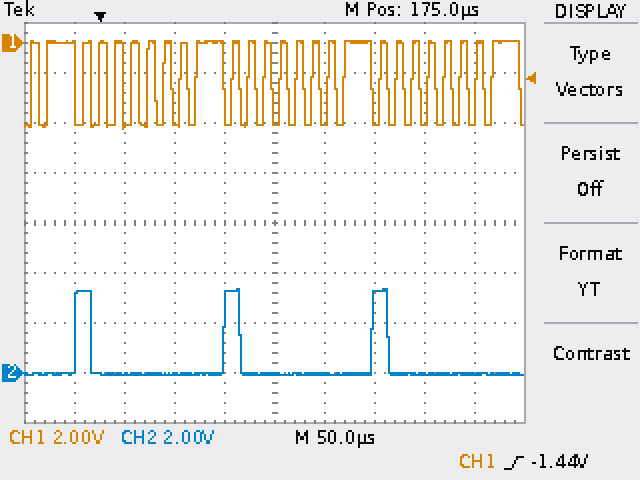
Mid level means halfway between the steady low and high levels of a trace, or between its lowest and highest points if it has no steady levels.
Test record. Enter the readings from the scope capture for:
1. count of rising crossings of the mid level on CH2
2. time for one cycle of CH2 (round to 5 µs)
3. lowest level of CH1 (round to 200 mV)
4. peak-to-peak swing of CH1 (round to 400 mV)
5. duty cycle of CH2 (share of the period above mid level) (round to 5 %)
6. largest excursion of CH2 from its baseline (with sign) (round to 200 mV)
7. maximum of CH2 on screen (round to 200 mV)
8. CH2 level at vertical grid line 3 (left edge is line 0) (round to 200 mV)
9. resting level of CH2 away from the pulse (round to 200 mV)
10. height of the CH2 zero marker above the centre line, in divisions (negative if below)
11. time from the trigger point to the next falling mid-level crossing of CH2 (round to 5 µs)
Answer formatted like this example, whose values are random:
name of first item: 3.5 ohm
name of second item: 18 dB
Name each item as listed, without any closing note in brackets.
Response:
count of rising crossings of the mid level on CH2: 3
time for one cycle of CH2: 150 µs
lowest level of CH1: -3.4 V
peak-to-peak swing of CH1: 3.6 V
duty cycle of CH2 (share of the period above mid level): 10 %
largest excursion of CH2 from its baseline (with sign): +3.4 V
maximum of CH2 on screen: 3.4 V
CH2 level at vertical grid line 3 (left edge is line 0): 0.0 V
resting level of CH2 away from the pulse: 0.0 V
height of the CH2 zero marker above the centre line, in divisions: -3.0 div
time from the trigger point to the next falling mid-level crossing of CH2: 140 µs
